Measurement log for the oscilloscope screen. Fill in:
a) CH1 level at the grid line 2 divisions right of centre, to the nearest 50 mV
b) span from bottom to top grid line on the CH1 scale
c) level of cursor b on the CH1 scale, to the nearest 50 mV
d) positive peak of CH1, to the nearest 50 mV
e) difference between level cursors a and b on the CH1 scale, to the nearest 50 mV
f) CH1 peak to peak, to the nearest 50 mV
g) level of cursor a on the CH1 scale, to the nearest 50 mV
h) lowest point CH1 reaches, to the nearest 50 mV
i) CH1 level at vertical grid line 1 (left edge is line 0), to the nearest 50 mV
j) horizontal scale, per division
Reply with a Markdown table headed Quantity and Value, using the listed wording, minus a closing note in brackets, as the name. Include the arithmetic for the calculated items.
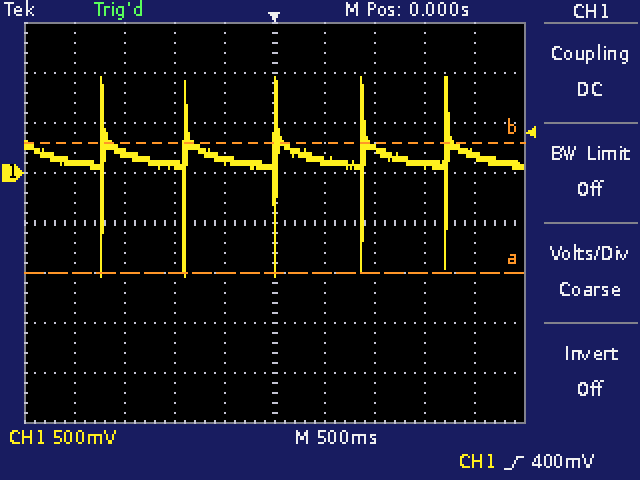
| Quantity | Value |
|---|---|
| CH1 level at the grid line 2 divisions right of centre, to the nearest 50 mV | 250 mV |
| span from bottom to top grid line on the CH1 scale | 4 V |
| level of cursor b on the CH1 scale, to the nearest 50 mV | 300 mV |
| positive peak of CH1, to the nearest 50 mV | 950 mV |
| difference between level cursors a and b on the CH1 scale, to the nearest 50 mV | 1.30 V |
| CH1 peak to peak, to the nearest 50 mV | 950 mV − (-1.05 V) = 2.00 V |
| level of cursor a on the CH1 scale, to the nearest 50 mV | -1.00 V |
| lowest point CH1 reaches, to the nearest 50 mV | -1.05 V |
| CH1 level at vertical grid line 1 (left edge is line 0), to the nearest 50 mV | 100 mV |
| horizontal scale, per division | 500 ms |
